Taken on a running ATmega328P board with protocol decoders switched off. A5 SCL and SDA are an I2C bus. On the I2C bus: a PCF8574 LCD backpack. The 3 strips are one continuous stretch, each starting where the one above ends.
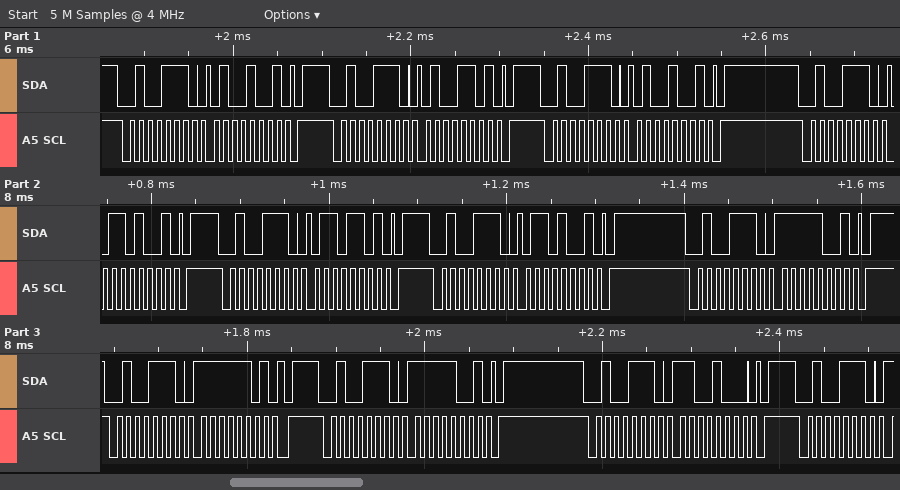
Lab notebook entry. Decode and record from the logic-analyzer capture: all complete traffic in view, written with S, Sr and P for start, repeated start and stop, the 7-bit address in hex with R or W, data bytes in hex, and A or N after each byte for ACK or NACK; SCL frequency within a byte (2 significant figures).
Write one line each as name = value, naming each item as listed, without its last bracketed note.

all complete traffic in view, written with S, Sr and P for start, repeated start and stop, the 7-bit address in hex with R or W, data bytes in hex, and A or N after each byte for ACK or NACK = S 27W A 49 A P S 27W A 4D A P S 27W A 49 A P S 27W A 69 A P S 27W A 6D A P S 27W A 69 A P S 27W A F9 A P S 27W A FD A P S 27W A F9 A P S 27W A C8 A P S 27W A
SCL frequency within a byte = 100 kHz
